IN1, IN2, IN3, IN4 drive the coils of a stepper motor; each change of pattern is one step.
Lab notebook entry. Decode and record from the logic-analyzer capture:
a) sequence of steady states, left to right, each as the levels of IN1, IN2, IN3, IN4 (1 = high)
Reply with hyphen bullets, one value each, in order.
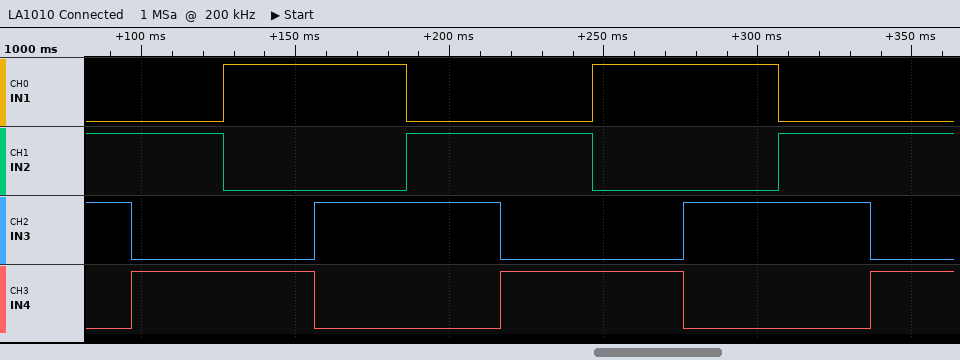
- 0110 0101 1001 1010 0110 0101 1001 1010 0110 0101
